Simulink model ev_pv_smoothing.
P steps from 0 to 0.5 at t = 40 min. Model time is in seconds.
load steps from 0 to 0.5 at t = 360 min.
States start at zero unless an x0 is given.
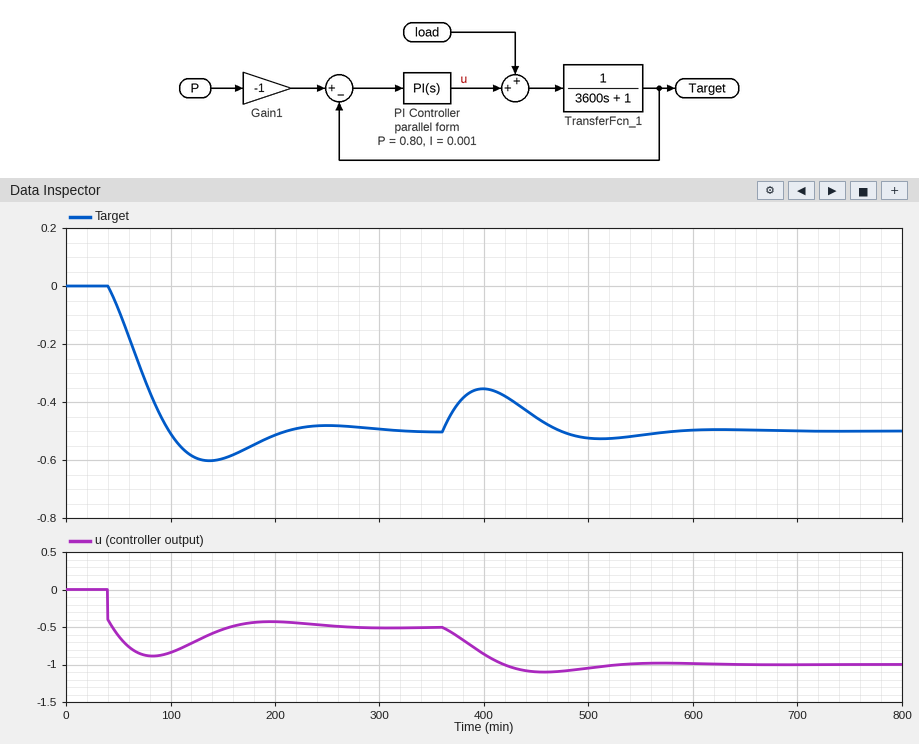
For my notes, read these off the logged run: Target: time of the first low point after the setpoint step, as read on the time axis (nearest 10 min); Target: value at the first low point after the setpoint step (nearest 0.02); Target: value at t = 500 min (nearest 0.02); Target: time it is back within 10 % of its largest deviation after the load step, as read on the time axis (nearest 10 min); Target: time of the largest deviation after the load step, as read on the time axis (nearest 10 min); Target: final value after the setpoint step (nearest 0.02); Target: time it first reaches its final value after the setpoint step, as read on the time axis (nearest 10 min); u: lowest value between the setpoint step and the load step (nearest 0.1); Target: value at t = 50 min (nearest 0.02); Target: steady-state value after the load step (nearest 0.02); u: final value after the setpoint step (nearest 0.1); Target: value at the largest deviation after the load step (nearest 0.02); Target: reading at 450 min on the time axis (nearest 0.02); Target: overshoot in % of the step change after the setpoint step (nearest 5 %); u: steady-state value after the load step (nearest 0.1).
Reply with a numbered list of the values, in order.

1. 140 min
2. -0.60
3. -0.52
4. 550 min
5. 400 min
6. -0.50
7. 100 min
8. -0.9
9. -0.08
10. -0.50
11. -0.5
12. -0.36
13. -0.46
14. 20 %
15. -1.0
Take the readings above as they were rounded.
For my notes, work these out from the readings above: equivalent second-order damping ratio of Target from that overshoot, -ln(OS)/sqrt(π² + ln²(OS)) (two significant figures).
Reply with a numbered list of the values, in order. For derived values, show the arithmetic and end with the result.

1. ln(0.2) = -1.609; 1.609 / sqrt(9.870 + 2.590) = 0.46
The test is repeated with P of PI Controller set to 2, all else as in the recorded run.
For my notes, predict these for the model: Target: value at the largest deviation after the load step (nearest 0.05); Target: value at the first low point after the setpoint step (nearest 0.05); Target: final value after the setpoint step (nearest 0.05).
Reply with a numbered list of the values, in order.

1. -0.40
2. -0.55
3. -0.50
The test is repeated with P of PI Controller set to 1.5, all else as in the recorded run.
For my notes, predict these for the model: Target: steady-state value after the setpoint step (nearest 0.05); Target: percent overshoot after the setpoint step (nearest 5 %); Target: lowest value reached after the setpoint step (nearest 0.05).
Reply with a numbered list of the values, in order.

1. -0.50
2. 10 %
3. -0.55
